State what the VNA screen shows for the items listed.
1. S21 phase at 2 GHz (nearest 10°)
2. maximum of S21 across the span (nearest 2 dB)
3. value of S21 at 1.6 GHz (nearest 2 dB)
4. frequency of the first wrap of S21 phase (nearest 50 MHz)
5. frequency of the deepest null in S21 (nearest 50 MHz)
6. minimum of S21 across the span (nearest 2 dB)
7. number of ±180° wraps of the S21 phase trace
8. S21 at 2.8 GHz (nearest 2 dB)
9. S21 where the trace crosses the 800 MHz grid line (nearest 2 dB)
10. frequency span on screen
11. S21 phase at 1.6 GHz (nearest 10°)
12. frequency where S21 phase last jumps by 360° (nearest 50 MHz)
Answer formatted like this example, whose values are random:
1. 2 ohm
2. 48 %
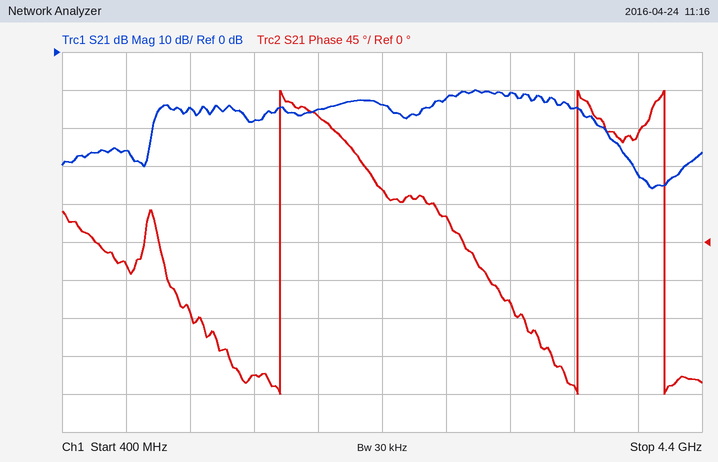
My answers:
1. 150°
2. -10 dB
3. -18 dB
4. 1.75 GHz
5. 4.10 GHz
6. -36 dB
7. 3
8. -12 dB
9. -26 dB
10. 4 GHz
11. -160°
12. 4.15 GHz
